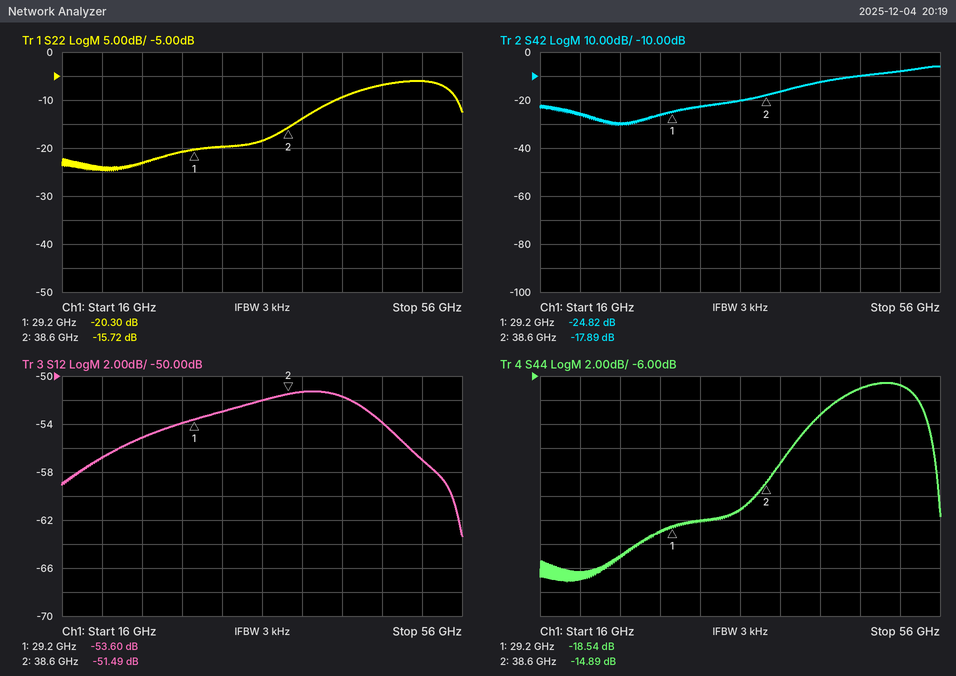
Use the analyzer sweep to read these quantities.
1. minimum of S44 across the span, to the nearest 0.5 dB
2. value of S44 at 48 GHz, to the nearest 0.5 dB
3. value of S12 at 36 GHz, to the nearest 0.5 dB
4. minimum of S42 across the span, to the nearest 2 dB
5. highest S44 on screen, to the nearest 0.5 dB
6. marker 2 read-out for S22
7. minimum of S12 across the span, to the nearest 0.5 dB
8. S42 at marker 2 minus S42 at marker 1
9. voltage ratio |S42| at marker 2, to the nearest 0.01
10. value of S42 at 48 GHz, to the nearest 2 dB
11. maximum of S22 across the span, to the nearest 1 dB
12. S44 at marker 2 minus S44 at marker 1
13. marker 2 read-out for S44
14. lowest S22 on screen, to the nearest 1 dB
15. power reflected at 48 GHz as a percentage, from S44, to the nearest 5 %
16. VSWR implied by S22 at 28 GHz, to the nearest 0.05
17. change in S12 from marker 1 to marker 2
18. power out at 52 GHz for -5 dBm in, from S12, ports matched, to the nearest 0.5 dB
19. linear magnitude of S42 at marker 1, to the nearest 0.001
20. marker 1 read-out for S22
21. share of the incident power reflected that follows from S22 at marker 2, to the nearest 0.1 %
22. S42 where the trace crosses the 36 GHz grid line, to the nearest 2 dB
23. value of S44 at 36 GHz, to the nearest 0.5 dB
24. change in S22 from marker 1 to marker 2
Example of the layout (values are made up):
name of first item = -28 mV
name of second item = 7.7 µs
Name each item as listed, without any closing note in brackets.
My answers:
minimum of S44 across the span, to the nearest 0.5 dB = -23.0 dB
value of S44 at 48 GHz, to the nearest 0.5 dB = -7.0 dB
value of S12 at 36 GHz, to the nearest 0.5 dB = -52.0 dB
minimum of S42 across the span, to the nearest 2 dB = -30 dB
highest S44 on screen, to the nearest 0.5 dB = -6.5 dB
marker 2 read-out for S22 = -15.72 dB
minimum of S12 across the span, to the nearest 0.5 dB = -63.5 dB
S42 at marker 2 minus S42 at marker 1 = 6.93 dB
voltage ratio |S42| at marker 2, to the nearest 0.01 = 0.13
value of S42 at 48 GHz, to the nearest 2 dB = -10 dB
maximum of S22 across the span, to the nearest 1 dB = -6 dB
S44 at marker 2 minus S44 at marker 1 = 3.65 dB
marker 2 read-out for S44 = -14.89 dB
lowest S22 on screen, to the nearest 1 dB = -25 dB
power reflected at 48 GHz as a percentage, from S44, to the nearest 5 % = 20 %
VSWR implied by S22 at 28 GHz, to the nearest 0.05 = 1.20
change in S12 from marker 1 to marker 2 = 2.11 dB
power out at 52 GHz for -5 dBm in, from S12, ports matched, to the nearest 0.5 dB = -62.0 dBm
linear magnitude of S42 at marker 1, to the nearest 0.001 = 0.057
marker 1 read-out for S22 = -20.30 dB
share of the incident power reflected that follows from S22 at marker 2, to the nearest 0.1 % = 2.7 %
S42 where the trace crosses the 36 GHz grid line, to the nearest 2 dB = -20 dB
value of S44 at 36 GHz, to the nearest 0.5 dB = -17.0 dB
change in S22 from marker 1 to marker 2 = 4.58 dB
